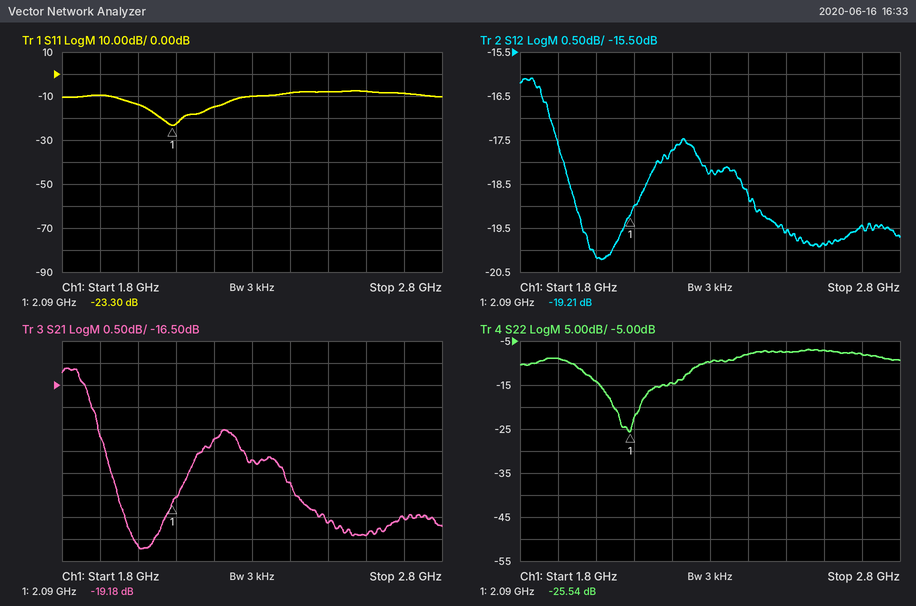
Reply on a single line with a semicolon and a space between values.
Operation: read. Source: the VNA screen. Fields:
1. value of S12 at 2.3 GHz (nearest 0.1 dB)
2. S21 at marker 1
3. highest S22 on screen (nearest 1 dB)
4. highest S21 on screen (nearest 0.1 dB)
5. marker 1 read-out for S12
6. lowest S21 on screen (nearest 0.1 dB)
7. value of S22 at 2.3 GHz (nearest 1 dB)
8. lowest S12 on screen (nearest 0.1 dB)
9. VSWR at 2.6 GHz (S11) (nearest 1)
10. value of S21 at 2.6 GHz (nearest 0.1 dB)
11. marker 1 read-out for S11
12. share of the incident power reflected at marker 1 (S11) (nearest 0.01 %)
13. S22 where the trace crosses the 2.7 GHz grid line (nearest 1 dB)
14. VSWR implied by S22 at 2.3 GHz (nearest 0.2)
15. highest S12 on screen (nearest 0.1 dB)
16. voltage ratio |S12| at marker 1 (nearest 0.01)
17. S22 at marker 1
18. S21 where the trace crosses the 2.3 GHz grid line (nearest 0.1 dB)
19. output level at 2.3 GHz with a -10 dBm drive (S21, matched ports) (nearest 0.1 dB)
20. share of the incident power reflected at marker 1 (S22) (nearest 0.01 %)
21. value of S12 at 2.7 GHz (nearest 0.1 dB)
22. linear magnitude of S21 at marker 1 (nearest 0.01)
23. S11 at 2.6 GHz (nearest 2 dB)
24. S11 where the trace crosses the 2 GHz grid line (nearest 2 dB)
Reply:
-18.2 dB; -19.18 dB; -7 dB; -16.1 dB; -19.21 dB; -20.2 dB; -10 dB; -20.2 dB; 2; -19.9 dB; -23.30 dB; 0.47 %; -8 dB; 2.0; -16.1 dB; 0.11; -25.54 dB; -18.2 dB; -28.2 dBm; 0.28 %; -19.4 dB; 0.11; -8 dB; -14 dB
